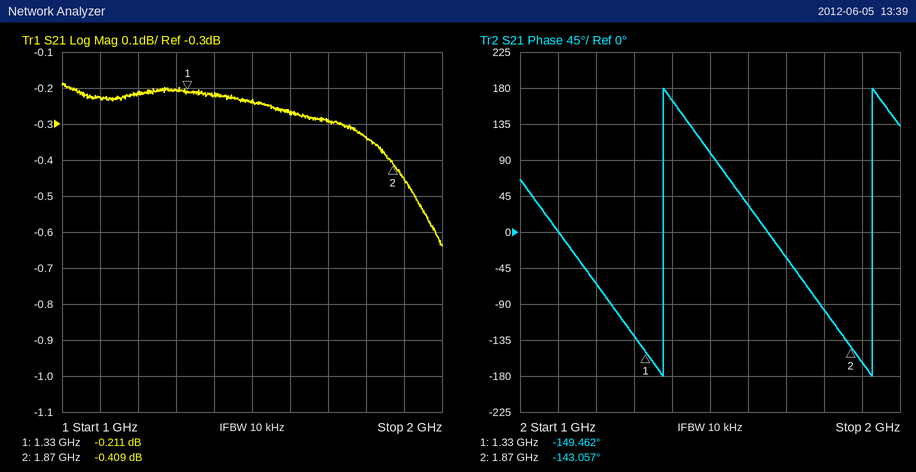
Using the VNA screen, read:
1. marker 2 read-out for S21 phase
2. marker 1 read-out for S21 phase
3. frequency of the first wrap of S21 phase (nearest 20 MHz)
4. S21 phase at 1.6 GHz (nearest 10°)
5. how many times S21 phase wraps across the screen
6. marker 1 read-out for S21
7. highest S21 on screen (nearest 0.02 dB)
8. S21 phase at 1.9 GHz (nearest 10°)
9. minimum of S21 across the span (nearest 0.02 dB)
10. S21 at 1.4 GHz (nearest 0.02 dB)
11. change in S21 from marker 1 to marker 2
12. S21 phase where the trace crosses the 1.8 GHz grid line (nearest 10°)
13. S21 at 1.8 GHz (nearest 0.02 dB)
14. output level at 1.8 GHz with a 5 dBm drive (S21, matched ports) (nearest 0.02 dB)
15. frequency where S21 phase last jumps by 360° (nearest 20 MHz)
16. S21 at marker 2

-143.057°
-149.462°
1.38 GHz
30°
2
-0.211 dB
-0.18 dB
-160°
-0.64 dB
-0.22 dB
-0.198 dB
-100°
-0.34 dB
4.66 dBm
1.92 GHz
-0.409 dB
